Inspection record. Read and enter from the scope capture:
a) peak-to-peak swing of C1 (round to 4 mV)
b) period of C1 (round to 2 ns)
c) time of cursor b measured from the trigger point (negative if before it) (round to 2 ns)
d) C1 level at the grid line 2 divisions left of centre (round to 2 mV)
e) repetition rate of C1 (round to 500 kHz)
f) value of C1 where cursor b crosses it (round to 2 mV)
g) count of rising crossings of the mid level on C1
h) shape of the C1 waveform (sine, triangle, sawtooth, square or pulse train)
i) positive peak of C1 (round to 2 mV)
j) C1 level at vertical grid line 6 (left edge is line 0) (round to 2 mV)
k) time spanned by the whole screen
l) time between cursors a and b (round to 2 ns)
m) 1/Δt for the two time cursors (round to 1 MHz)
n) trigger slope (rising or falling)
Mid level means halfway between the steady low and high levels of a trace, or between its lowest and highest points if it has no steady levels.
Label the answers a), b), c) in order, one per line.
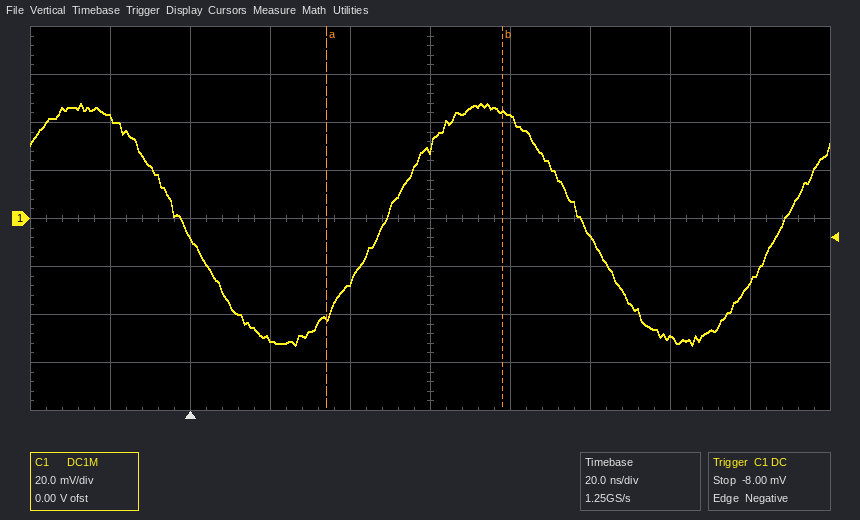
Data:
a) 100 mV
b) 100 ns
c) +78 ns
d) -50 mV
e) 10.0 MHz
f) 44 mV
g) 2
h) sine
i) 48 mV
j) 42 mV
k) 200 ns
l) 44 ns
m) 23 MHz
n) falling
